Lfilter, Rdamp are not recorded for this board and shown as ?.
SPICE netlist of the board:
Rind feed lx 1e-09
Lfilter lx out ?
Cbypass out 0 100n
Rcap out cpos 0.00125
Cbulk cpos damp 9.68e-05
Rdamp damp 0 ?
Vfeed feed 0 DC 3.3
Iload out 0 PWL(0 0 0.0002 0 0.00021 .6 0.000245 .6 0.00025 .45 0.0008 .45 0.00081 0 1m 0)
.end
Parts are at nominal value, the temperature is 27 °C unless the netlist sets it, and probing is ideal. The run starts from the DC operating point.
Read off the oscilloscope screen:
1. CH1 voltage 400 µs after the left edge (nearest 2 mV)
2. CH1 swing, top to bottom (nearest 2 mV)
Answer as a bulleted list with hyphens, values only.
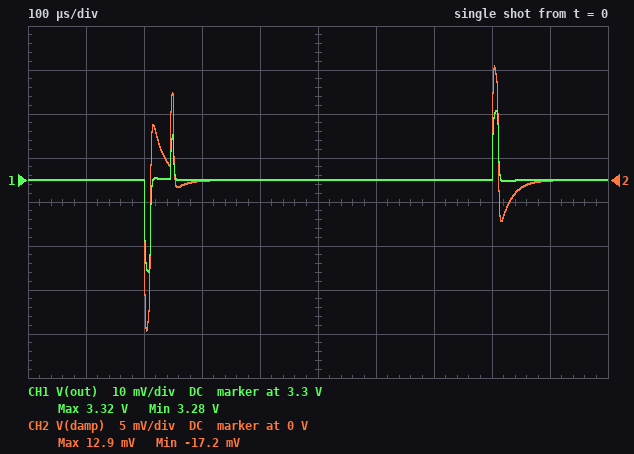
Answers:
- 3.300 V
- 36 mV
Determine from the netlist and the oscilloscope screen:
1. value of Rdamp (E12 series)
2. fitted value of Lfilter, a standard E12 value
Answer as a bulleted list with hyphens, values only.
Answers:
- 0.22 Ω
- 330 nH
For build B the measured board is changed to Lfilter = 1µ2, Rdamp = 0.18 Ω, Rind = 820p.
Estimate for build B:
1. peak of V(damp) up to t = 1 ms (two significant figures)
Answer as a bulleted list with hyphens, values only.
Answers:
- 36 mV
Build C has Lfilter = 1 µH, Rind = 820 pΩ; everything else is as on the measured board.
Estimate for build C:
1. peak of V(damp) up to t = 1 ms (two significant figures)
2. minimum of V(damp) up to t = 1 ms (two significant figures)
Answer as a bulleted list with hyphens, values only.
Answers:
- 34 mV
- -45 mV
